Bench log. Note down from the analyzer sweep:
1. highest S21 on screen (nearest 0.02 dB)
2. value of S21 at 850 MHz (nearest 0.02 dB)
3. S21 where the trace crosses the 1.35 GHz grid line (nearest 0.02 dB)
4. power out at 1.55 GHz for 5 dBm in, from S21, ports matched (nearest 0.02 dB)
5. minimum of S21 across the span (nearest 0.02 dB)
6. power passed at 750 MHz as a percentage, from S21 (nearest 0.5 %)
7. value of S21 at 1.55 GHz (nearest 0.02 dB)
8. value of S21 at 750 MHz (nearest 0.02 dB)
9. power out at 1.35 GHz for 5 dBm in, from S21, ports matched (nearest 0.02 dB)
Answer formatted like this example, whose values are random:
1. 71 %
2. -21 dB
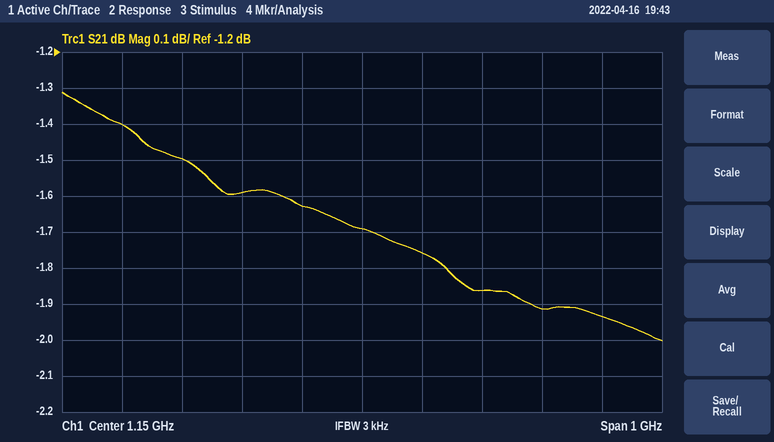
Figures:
1. -1.32 dB
2. -1.50 dB
3. -1.86 dB
4. 3.06 dBm
5. -2.00 dB
6. 72.5 %
7. -1.94 dB
8. -1.40 dB
9. 3.14 dBm
